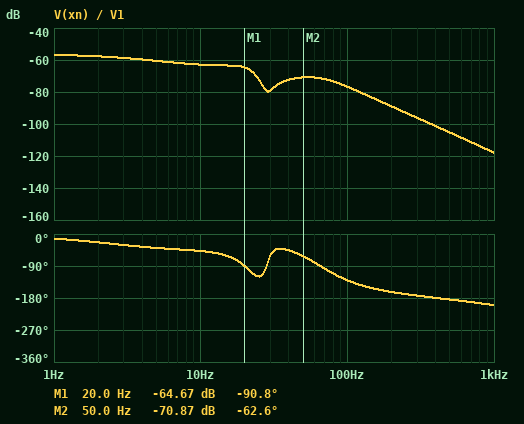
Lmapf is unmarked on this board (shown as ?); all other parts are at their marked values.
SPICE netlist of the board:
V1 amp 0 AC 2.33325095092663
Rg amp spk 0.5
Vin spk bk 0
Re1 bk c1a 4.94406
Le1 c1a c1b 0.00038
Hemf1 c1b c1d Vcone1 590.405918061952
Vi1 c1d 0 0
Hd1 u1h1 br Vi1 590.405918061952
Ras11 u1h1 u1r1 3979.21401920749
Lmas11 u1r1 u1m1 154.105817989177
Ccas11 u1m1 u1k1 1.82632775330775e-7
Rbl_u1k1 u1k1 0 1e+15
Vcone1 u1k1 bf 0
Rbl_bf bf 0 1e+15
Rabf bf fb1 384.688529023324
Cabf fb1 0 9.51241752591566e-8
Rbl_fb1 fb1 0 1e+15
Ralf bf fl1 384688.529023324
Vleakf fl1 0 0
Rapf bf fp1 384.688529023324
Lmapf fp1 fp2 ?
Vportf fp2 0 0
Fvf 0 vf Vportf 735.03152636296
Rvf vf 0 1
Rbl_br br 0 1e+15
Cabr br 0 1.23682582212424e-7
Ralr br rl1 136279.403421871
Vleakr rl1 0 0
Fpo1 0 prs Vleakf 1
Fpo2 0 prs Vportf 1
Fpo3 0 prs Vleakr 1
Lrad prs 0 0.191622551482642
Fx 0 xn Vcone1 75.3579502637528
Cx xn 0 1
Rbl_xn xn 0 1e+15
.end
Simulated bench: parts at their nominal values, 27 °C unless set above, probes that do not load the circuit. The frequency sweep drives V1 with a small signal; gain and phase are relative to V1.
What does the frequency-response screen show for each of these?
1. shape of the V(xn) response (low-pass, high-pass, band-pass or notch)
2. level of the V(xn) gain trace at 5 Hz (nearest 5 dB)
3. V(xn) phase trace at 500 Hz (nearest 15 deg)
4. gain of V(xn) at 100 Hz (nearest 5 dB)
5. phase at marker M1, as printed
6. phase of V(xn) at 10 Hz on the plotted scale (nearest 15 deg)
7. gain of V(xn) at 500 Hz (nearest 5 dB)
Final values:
low-pass
-60 dB
-180 deg
-75 dB
-90.8 deg
-45 deg
-105 dB
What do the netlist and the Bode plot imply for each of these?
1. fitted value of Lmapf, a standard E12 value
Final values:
330 H
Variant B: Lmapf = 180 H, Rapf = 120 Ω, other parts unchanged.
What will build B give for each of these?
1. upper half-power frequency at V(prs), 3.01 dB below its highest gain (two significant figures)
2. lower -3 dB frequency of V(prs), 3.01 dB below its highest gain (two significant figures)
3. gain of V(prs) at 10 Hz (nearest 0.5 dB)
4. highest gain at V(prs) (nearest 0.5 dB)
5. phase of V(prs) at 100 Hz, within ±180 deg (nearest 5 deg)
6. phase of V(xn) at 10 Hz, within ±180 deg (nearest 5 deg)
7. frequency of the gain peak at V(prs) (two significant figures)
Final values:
59 Hz
27 Hz
-45.5 dB
-20.5 dB
-140 deg
-45 deg
35 Hz
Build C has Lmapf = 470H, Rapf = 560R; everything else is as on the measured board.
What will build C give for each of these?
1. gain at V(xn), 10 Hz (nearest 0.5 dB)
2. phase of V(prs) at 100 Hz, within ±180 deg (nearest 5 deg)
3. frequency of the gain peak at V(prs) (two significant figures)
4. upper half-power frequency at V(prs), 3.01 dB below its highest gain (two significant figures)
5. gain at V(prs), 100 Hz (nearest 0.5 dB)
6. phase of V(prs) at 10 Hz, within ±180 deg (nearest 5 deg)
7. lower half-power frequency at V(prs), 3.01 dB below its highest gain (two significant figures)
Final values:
-62.5 dB
-165 deg
20 Hz
36 Hz
-39.0 dB
160 deg
16 Hz
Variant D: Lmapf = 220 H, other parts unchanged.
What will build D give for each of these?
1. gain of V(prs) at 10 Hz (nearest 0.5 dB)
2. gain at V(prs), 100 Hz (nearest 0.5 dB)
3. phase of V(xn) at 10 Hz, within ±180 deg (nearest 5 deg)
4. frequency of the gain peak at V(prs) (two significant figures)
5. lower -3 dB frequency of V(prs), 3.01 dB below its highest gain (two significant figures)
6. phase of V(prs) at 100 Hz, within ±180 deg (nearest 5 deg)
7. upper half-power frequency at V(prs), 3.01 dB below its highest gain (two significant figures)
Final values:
-45.0 dB
-33.5 dB
-45 deg
31 Hz
24 Hz
-145 deg
54 Hz
